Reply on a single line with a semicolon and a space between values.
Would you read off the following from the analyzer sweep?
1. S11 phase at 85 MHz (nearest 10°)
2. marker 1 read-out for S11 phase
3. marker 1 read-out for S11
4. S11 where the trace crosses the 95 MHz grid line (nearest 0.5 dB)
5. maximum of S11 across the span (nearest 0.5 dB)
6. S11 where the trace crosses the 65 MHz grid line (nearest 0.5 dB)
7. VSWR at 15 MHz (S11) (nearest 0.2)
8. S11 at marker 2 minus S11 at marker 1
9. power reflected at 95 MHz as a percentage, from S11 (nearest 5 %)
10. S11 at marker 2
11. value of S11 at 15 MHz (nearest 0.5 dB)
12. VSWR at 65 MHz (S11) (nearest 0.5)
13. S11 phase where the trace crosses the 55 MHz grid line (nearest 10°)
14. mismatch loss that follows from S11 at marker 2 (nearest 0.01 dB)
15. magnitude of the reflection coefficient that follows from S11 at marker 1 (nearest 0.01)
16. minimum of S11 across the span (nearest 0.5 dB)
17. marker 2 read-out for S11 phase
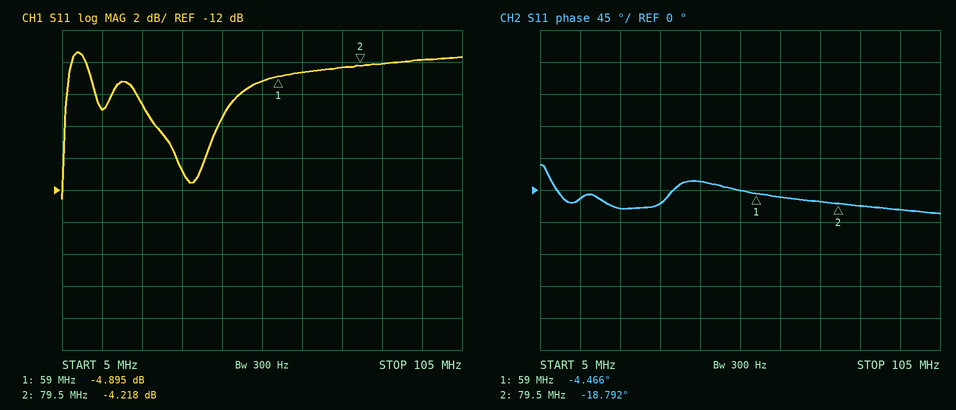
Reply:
-20°; -4.466°; -4.895 dB; -4.0 dB; -3.5 dB; -4.5 dB; 2.6; 0.677 dB; 40 %; -4.218 dB; -7.0 dB; 4.0; 0°; 2.07 dB; 0.57; -12.5 dB; -18.792°
